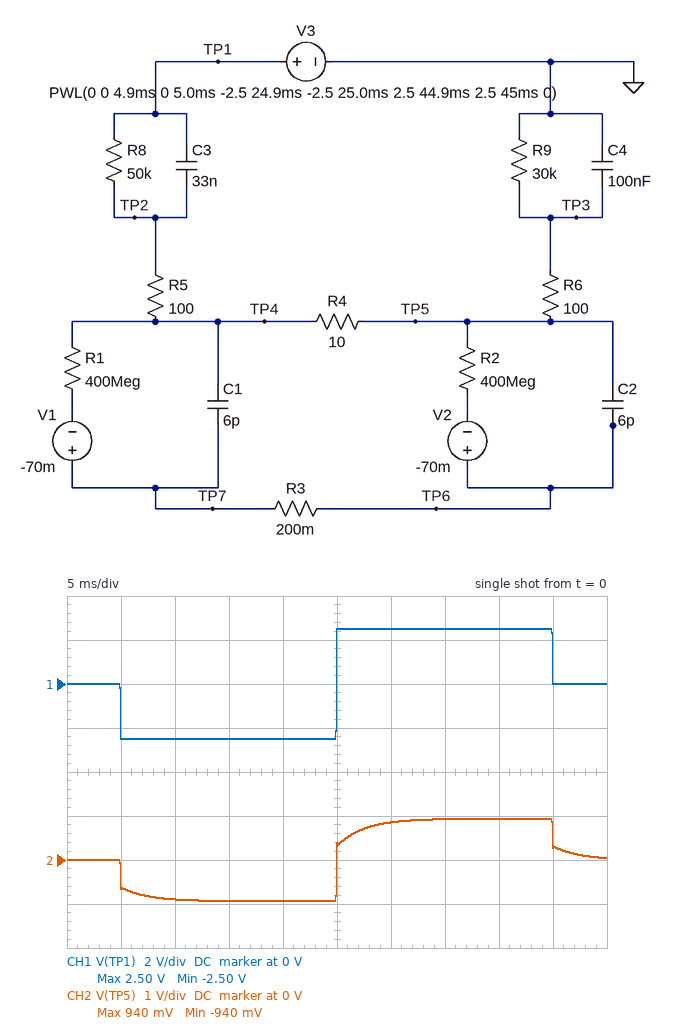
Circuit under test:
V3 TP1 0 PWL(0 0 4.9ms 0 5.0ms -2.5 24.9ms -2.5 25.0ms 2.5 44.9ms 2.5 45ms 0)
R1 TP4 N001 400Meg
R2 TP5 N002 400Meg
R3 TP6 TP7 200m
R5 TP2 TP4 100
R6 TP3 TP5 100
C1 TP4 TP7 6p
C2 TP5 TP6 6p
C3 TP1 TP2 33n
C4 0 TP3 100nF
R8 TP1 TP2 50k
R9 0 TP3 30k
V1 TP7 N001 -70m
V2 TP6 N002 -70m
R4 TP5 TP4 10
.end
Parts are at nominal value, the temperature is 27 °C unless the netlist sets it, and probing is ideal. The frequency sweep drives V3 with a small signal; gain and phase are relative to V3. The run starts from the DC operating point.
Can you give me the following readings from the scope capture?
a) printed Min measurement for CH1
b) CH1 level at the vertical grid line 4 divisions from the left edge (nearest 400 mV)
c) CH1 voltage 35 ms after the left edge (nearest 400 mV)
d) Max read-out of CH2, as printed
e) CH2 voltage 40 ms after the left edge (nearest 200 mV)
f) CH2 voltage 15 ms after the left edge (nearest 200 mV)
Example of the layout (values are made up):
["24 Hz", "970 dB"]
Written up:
["-2.50 V", "-2.4 V", "2.4 V", "940 mV", "1.0 V", "-1.0 V"]
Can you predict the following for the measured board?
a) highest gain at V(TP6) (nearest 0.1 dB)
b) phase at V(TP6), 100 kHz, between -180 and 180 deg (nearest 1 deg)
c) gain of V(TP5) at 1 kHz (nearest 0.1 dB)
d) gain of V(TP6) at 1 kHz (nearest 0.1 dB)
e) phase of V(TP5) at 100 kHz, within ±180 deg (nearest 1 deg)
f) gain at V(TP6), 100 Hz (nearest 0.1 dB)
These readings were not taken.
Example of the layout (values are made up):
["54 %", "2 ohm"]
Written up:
["-6.0 dB", "8 deg", "-12.1 dB", "-12.1 dB", "8 deg", "-10.7 dB"]
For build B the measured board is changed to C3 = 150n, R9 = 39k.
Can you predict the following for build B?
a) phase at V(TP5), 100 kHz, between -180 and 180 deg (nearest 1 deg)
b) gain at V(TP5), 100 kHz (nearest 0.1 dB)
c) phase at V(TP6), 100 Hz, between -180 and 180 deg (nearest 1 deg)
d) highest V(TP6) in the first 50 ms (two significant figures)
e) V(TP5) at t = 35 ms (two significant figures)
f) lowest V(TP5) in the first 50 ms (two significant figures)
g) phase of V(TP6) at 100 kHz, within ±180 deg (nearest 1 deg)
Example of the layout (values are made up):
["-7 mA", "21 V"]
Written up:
["-2 deg", "-6.4 dB", "4 deg", "1.8 V", "1.2 V", "-1.5 V", "-1 deg"]
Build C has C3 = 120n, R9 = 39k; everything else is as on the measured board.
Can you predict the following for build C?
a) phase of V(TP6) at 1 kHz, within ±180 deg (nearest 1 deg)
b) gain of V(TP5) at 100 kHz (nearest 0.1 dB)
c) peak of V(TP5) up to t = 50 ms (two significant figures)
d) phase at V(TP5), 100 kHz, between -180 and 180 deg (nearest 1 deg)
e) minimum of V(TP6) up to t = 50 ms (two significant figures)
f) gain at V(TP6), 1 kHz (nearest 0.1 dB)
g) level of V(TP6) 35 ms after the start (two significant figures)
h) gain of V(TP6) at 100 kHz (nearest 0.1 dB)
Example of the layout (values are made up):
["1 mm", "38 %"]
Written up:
["0 deg", "-6.4 dB", "1.6 V", "-1 deg", "-1.4 V", "-5.3 dB", "1.1 V", "-6.0 dB"]
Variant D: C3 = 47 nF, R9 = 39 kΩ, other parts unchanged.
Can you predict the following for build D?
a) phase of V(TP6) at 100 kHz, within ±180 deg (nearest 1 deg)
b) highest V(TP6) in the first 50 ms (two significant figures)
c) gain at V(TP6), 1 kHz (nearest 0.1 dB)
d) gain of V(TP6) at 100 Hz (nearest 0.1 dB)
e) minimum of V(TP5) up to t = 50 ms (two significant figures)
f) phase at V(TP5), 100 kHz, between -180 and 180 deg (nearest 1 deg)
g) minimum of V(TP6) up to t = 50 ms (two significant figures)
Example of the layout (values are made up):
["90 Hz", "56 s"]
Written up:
["5 deg", "1.0 V", "-9.9 dB", "-9.2 dB", "-1.1 V", "4 deg", "-1.2 V"]
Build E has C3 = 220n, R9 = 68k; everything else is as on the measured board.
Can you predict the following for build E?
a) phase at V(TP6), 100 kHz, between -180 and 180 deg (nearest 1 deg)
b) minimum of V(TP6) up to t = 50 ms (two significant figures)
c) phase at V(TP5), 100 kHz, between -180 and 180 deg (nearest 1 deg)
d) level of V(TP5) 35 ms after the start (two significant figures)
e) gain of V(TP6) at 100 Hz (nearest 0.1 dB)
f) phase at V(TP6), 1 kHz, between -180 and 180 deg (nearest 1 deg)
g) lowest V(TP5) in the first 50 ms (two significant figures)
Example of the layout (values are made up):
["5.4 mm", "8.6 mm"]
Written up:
["-2 deg", "-1.8 V", "-3 deg", "1.6 V", "-3.3 dB", "-1 deg", "-1.7 V"]
